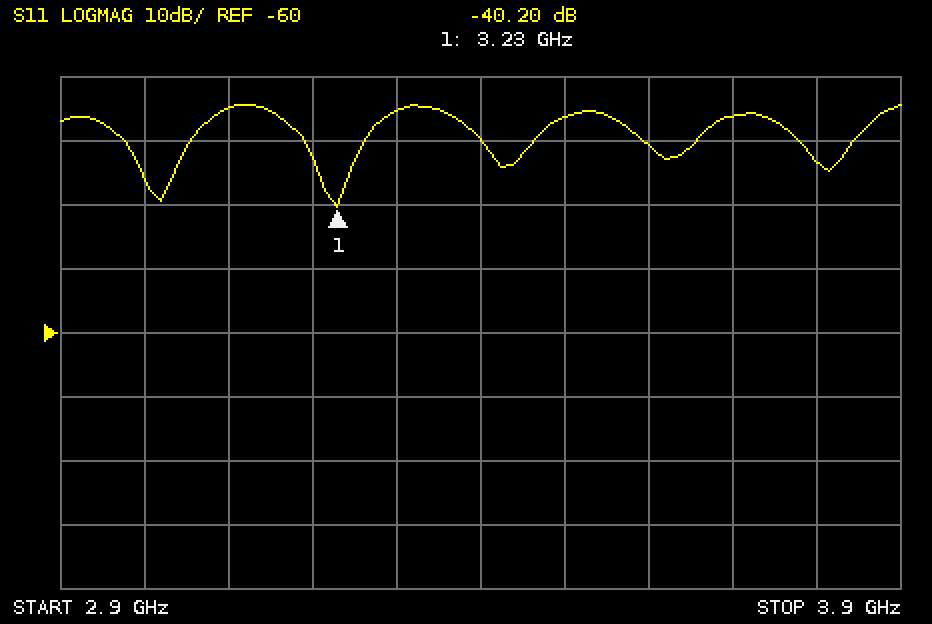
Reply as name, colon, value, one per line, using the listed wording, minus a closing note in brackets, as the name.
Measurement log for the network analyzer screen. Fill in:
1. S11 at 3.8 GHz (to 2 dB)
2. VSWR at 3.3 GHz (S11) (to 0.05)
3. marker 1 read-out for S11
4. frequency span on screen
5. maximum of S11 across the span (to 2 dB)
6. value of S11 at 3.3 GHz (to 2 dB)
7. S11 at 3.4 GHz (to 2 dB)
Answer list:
S11 at 3.8 GHz: -34 dB
VSWR at 3.3 GHz (S11): 1.10
marker 1 read-out for S11: -40.20 dB
frequency span on screen: 1 GHz
maximum of S11 across the span: -24 dB
value of S11 at 3.3 GHz: -26 dB
S11 at 3.4 GHz: -30 dB
